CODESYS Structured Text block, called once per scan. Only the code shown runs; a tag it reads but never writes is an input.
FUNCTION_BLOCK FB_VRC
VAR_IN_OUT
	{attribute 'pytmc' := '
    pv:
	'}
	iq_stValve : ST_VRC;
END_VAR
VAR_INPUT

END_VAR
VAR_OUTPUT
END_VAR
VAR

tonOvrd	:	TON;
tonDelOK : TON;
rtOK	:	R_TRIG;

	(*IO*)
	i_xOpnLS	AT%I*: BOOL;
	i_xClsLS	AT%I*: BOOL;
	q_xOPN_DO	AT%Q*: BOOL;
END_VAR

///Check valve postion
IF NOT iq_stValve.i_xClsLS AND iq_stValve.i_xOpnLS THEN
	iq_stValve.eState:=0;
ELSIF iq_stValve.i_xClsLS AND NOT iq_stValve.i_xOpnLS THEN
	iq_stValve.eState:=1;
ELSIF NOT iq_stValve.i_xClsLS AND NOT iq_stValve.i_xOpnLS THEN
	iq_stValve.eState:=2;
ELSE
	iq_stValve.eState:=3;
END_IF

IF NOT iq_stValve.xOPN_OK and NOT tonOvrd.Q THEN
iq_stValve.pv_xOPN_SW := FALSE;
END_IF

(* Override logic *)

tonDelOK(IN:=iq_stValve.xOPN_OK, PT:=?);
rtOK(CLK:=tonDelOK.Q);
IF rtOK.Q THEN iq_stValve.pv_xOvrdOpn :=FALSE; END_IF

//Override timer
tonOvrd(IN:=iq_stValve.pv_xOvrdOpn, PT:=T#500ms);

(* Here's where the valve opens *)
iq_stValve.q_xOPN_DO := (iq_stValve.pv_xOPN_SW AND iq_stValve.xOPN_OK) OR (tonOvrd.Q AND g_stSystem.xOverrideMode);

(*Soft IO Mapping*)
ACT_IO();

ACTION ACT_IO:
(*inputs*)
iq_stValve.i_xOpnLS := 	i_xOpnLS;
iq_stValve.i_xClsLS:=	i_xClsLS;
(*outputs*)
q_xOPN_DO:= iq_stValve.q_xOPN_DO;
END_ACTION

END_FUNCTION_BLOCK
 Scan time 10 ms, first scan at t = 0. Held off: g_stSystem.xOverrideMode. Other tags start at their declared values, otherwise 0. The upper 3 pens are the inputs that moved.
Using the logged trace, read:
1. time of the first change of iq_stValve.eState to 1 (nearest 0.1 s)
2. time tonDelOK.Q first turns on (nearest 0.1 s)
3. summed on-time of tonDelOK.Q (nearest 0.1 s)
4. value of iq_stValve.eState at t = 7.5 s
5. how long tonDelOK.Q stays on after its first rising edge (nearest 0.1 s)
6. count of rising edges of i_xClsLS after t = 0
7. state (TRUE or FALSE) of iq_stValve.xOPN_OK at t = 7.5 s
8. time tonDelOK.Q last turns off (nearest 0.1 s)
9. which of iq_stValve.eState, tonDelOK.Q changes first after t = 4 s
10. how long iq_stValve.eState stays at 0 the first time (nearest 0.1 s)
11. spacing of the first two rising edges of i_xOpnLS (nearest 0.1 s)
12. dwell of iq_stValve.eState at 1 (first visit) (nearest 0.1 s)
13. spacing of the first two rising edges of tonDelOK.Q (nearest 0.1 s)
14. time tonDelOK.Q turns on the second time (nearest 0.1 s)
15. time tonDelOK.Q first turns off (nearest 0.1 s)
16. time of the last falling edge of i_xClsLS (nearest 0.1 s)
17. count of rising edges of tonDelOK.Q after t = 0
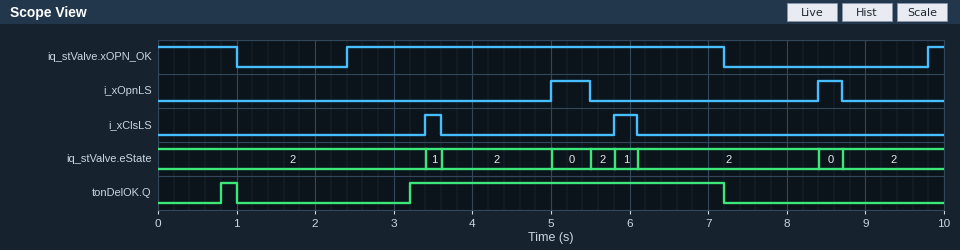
3.4 s
0.8 s
4.2 s
2
0.2 s
2
FALSE
7.2 s
iq_stValve.eState
0.5 s
3.4 s
0.2 s
2.4 s
3.2 s
1.0 s
6.1 s
2
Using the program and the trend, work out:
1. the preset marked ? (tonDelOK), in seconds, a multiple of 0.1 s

0.8 s
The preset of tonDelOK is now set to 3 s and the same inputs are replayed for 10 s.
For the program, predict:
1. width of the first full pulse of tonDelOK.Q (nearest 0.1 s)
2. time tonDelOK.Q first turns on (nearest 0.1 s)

1.8 s
5.4 s
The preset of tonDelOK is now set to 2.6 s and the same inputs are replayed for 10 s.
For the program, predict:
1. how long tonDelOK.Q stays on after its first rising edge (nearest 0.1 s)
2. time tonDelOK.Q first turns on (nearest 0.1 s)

2.2 s
5.0 s
